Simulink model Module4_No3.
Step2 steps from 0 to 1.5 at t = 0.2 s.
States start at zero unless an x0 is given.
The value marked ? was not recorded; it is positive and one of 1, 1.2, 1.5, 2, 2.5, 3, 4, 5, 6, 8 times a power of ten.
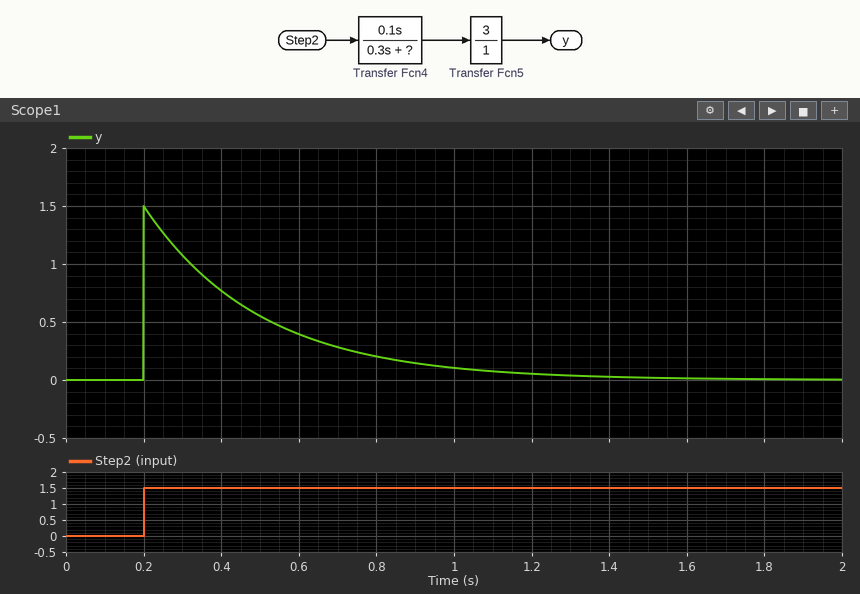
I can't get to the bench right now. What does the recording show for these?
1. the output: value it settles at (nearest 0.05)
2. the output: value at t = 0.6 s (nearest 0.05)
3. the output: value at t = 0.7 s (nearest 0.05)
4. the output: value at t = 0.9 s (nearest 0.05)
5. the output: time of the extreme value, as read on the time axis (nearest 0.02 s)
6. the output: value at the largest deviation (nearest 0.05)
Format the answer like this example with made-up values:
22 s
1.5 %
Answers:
0.00
0.40
0.30
0.15
0.20 s
1.50
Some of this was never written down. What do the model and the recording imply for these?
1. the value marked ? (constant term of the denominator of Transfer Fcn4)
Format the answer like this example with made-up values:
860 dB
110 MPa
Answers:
1
